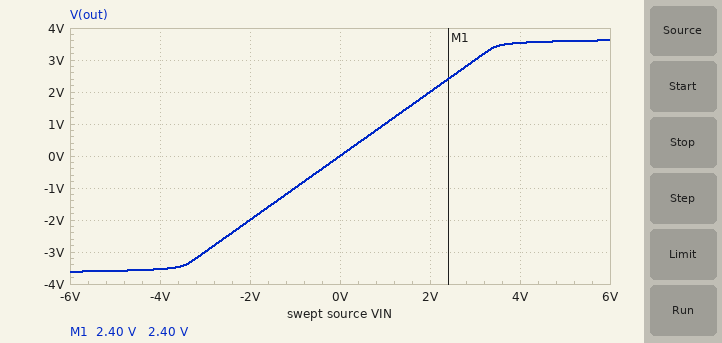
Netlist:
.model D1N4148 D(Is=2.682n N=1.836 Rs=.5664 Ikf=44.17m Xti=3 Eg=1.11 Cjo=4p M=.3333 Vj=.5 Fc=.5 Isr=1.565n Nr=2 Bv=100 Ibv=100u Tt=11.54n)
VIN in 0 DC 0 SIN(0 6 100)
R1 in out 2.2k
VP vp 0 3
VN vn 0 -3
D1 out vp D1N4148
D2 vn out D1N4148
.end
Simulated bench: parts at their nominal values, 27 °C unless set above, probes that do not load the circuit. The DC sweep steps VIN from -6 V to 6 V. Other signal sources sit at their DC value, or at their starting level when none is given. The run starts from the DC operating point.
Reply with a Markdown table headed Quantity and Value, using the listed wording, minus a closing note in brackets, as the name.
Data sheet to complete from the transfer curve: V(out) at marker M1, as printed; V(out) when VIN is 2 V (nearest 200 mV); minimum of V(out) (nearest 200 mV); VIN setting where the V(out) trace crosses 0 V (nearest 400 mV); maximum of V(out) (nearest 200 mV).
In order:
| Quantity | Value |
|---|---|
| V(out) at marker M1, as printed | 2.40 V |
| V(out) when VIN is 2 V | 2.0 V |
| minimum of V(out) | -3.6 V |
| VIN setting where the V(out) trace crosses 0 V | 0 V |
| maximum of V(out) | 3.6 V |
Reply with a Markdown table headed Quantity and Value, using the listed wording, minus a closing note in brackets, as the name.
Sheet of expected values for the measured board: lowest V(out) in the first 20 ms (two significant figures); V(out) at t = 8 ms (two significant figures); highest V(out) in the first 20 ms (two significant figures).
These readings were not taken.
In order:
| Quantity | Value |
|---|---|
| lowest V(out) in the first 20 ms | -3.6 V |
| V(out) at t = 8 ms | -3.6 V |
| highest V(out) in the first 20 ms | 3.6 V |
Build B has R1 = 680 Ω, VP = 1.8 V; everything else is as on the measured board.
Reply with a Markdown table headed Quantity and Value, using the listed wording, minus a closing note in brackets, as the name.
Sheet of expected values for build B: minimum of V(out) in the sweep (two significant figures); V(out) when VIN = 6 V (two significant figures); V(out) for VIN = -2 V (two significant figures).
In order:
| Quantity | Value |
|---|---|
| minimum of V(out) in the sweep | -3.7 V |
| V(out) when VIN = 6 V | 2.5 V |
| V(out) for VIN = -2 V | -2.0 V |
